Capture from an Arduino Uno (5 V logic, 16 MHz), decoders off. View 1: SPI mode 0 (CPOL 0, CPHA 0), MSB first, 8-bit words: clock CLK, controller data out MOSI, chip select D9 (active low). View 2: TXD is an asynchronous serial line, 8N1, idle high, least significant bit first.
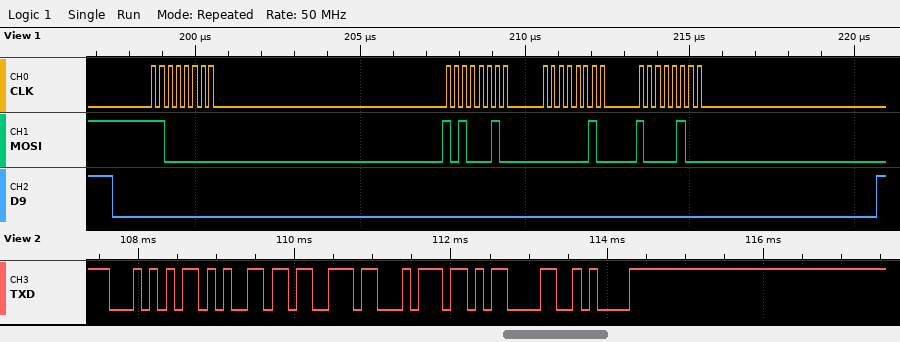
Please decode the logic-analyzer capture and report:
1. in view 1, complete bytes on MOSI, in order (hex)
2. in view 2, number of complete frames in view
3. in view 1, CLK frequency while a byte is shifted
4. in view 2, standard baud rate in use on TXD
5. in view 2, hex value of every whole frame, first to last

C0 A2 02 84
6
4 MHz
9600 baud
0x54 0x65 0x73 0x74 0x0D 0x0A
